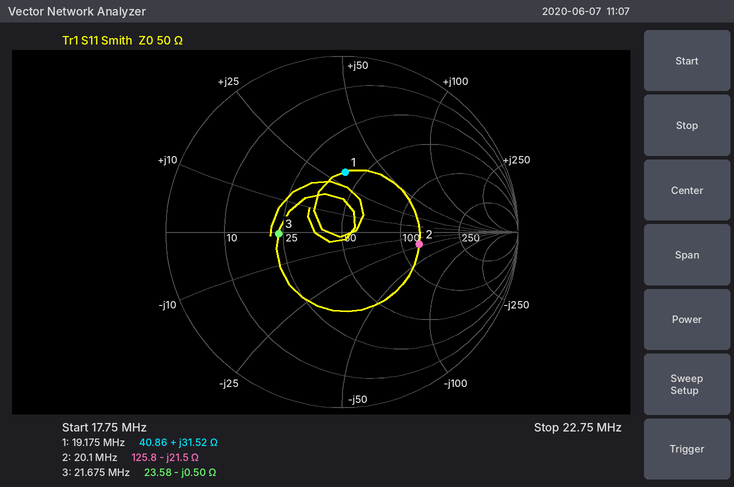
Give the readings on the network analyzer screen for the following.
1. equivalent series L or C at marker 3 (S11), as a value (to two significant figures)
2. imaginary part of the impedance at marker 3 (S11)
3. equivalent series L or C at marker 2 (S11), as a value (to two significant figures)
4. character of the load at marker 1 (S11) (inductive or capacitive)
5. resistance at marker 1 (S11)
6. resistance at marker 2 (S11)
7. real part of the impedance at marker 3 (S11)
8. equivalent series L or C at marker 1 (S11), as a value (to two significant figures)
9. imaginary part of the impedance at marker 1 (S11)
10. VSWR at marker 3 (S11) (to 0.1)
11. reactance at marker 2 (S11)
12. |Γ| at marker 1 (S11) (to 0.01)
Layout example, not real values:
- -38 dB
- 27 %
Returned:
- 15 nF
- -0.50 Ω
- 370 pF
- inductive
- 40.86 Ω
- 125.8 Ω
- 23.58 Ω
- 260 nH
- +31.52 Ω
- 2.1
- -21.5 Ω
- 0.34
